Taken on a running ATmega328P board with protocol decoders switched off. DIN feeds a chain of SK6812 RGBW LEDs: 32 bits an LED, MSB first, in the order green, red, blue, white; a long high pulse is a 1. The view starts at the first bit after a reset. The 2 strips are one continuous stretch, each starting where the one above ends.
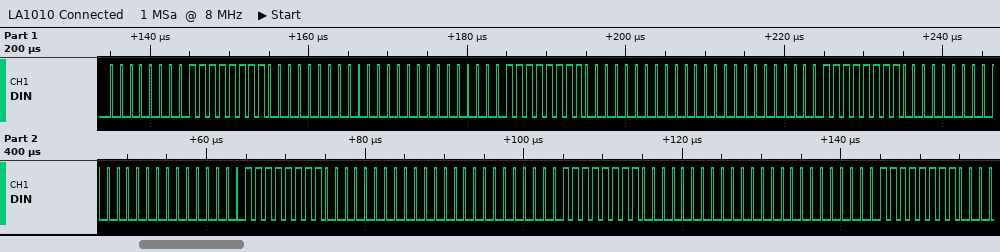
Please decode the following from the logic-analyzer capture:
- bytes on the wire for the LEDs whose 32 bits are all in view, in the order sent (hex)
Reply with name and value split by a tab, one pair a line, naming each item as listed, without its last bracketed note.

bytes on the wire for the LEDs whose 32 bits are all in view, in the order sent	00 FF 00 00 00 FF 00 00 00 FF 00 00 00 FF 00 00 00 FF 00 00
